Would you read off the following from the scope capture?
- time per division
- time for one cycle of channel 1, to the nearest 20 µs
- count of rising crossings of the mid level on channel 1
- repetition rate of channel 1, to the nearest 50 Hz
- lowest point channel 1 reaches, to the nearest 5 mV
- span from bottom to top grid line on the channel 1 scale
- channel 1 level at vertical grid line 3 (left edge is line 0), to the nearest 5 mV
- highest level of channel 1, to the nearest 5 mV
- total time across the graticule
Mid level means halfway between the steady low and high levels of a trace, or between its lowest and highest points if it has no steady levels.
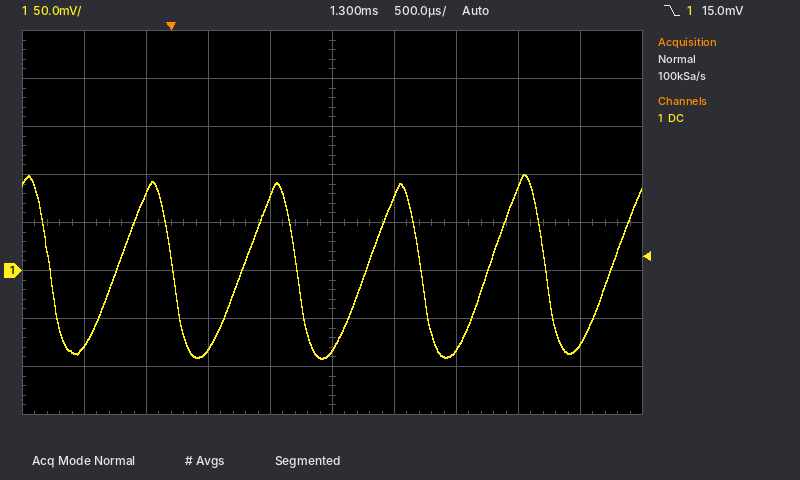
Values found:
500 µs
1.00 ms
5
1.00 kHz
-90 mV
400 mV
-80 mV
100 mV
5 ms
